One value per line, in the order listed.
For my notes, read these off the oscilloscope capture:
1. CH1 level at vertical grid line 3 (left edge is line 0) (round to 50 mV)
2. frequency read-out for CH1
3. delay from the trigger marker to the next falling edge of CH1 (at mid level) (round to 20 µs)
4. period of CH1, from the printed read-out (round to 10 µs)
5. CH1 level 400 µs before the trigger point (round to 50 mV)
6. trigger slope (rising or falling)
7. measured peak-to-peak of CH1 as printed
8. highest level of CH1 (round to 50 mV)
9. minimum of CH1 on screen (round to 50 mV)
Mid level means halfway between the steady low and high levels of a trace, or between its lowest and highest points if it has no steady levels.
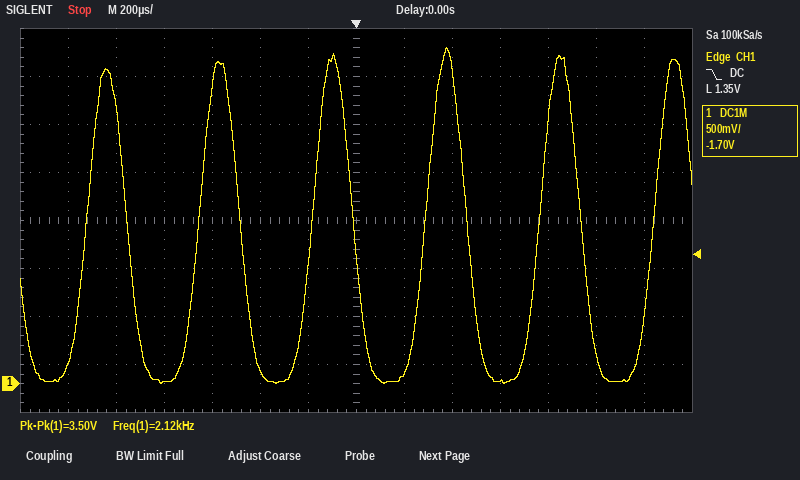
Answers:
0 mV
2.12 kHz
460 µs
470 µs
150 mV
falling
3.50 V
3.50 V
0 mV
